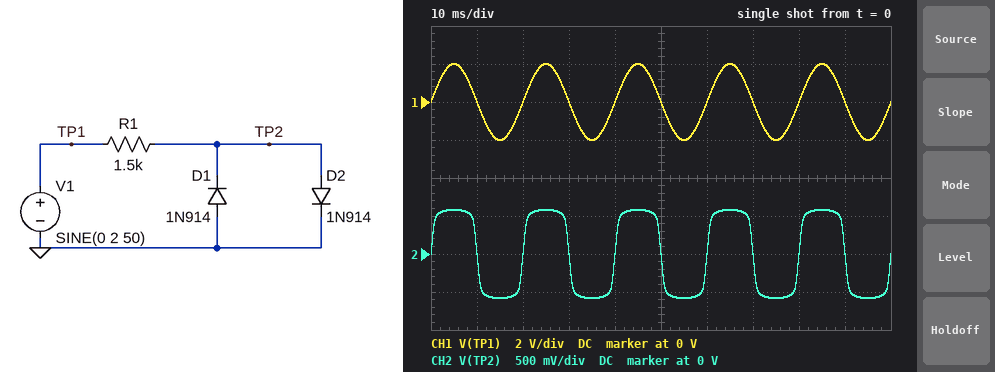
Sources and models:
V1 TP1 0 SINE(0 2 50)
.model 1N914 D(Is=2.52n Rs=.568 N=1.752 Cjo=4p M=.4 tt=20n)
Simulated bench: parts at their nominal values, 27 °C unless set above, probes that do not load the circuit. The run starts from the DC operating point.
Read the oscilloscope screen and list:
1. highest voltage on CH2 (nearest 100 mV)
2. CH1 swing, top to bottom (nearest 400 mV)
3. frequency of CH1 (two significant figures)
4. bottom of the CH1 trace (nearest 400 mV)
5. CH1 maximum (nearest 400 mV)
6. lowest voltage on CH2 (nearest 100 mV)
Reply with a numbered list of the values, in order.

1. 600 mV
2. 4.0 V
3. 50 Hz
4. -2.0 V
5. 2.0 V
6. -600 mV
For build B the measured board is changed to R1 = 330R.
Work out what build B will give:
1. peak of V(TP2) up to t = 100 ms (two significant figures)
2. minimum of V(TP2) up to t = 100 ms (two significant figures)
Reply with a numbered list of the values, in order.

1. 650 mV
2. -650 mV
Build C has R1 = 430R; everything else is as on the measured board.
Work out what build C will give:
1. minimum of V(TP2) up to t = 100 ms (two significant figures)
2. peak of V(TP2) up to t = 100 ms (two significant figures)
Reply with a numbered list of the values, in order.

1. -640 mV
2. 640 mV
